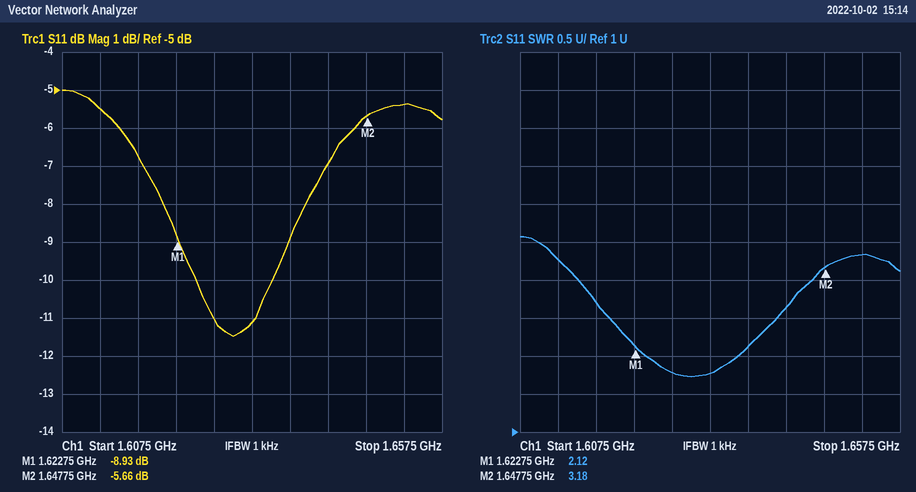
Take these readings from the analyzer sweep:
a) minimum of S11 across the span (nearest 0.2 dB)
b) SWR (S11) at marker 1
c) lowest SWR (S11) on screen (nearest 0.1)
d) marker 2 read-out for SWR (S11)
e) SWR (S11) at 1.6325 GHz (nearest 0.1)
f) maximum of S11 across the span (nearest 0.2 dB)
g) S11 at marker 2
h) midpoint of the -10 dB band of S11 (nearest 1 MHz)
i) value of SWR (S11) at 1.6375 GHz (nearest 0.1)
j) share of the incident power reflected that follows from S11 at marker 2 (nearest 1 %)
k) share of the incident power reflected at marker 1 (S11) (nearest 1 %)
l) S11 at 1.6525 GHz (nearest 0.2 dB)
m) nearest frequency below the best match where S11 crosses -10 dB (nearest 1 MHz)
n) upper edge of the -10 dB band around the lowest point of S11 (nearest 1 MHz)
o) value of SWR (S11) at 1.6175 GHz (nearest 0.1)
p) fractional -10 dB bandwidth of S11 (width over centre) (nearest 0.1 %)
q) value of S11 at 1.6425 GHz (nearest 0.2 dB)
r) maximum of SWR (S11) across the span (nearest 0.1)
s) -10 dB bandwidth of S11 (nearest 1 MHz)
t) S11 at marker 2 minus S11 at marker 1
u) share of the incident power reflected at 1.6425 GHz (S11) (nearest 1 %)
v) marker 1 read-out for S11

-11.4 dB
2.12
1.7
3.18
1.8
-5.0 dB
-5.66 dB
1.630 GHz
2.1
27 %
13 %
-5.4 dB
1.625 GHz
1.635 GHz
2.7
0.6 %
-7.0 dB
3.6
10 MHz
3.27 dB
20 %
-8.93 dB
